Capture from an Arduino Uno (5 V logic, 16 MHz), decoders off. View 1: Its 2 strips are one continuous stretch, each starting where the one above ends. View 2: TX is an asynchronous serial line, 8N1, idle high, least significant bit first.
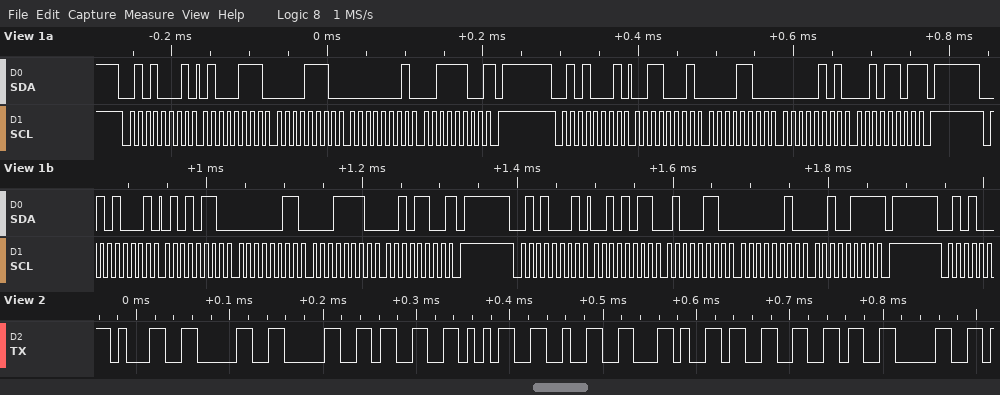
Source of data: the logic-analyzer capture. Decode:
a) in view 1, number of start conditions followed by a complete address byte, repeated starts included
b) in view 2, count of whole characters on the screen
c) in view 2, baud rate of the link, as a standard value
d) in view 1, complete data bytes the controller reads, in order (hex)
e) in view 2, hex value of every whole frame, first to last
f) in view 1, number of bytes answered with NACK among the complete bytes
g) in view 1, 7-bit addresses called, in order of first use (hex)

4
10
115200 baud
47 0E 01 3C 31 0C 05 2D 56 03 1E 2C 2B 46 02 27
31 30 30 33 35 32 2C 33 36 30
4
0x28
